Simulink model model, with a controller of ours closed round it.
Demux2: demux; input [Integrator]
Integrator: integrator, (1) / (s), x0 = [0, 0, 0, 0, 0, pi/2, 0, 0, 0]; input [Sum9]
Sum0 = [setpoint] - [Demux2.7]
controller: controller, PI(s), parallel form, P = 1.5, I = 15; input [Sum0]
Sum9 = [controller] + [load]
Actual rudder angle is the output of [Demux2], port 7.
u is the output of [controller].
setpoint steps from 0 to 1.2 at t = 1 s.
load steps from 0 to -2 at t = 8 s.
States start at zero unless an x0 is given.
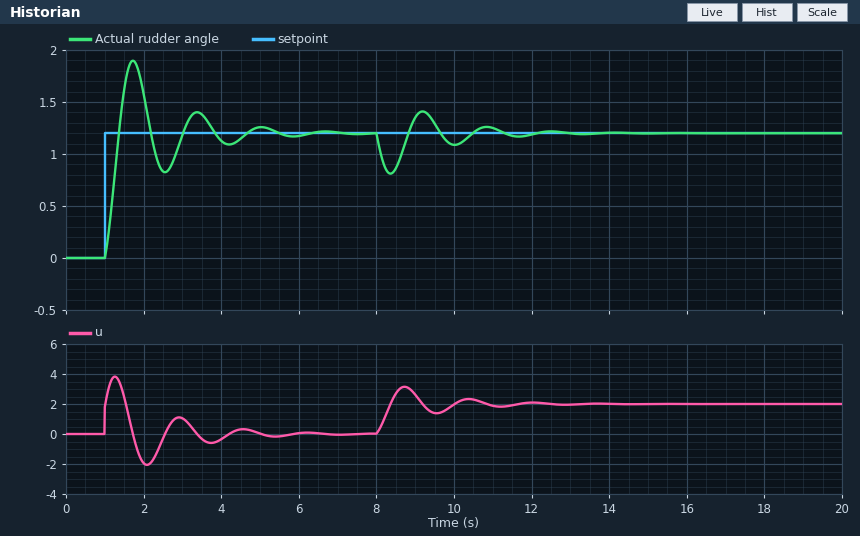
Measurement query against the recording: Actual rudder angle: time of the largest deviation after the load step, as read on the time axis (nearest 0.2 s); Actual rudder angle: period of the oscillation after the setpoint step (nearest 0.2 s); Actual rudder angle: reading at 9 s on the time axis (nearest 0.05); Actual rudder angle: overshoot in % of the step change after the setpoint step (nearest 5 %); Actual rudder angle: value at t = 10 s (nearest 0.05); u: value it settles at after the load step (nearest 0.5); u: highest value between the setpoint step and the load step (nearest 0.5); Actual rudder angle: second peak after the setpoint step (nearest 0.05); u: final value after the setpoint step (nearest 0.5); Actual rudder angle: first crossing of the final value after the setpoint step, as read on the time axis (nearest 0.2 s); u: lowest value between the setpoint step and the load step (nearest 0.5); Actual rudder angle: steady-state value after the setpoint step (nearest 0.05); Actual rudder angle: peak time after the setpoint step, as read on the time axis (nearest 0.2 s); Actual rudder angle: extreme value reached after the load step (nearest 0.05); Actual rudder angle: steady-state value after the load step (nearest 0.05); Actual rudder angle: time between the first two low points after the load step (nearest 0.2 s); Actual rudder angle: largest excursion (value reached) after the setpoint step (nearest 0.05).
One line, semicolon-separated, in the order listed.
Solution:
8.4 s; 1.6 s; 1.35; 60 %; 1.10; 2.0; 4.0; 1.40; 0.0; 1.4 s; -2.0; 1.20; 1.8 s; 0.80; 1.20; 1.6 s; 1.90
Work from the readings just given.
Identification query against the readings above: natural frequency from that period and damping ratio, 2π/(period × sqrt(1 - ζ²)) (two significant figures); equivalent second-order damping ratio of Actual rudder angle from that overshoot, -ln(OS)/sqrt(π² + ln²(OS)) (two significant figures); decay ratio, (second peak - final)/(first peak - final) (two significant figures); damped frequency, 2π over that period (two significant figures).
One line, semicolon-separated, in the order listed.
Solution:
4.0 rad/s; 0.16; 0.29; 3.9 rad/s
